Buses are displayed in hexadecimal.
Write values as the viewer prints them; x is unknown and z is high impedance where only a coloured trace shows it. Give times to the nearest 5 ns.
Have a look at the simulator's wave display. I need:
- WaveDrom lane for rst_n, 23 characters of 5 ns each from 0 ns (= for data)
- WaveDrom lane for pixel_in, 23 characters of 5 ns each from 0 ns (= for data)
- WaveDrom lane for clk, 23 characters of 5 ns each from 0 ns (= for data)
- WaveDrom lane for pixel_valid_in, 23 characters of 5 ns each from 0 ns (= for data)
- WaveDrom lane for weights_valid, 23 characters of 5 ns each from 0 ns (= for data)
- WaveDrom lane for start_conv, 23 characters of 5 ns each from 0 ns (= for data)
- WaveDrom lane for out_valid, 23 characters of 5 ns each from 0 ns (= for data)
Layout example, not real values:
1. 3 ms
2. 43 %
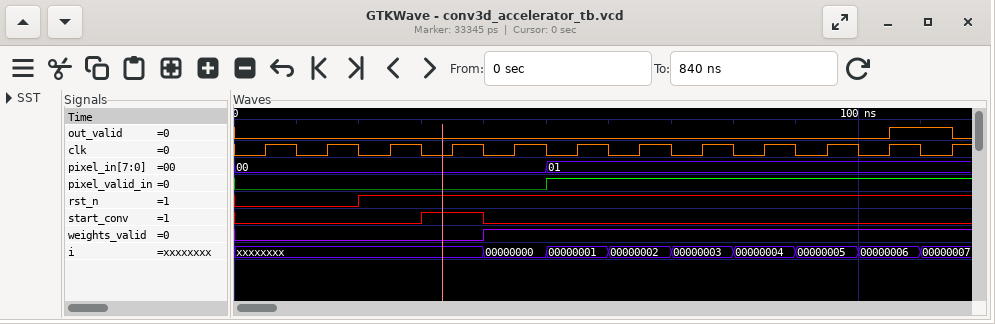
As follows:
1. {name: 'rst_n', wave: '0...1..................'}
2. {name: 'pixel_in', wave: '=.........=............', data: '00 01'}
3. {name: 'clk', wave: '01010101010101010101010'}
4. {name: 'pixel_valid_in', wave: '0.........1............'}
5. {name: 'weights_valid', wave: '0.......1..............'}
6. {name: 'start_conv', wave: '0.....1.0..............'}
7. {name: 'out_valid', wave: '0....................1.'}
